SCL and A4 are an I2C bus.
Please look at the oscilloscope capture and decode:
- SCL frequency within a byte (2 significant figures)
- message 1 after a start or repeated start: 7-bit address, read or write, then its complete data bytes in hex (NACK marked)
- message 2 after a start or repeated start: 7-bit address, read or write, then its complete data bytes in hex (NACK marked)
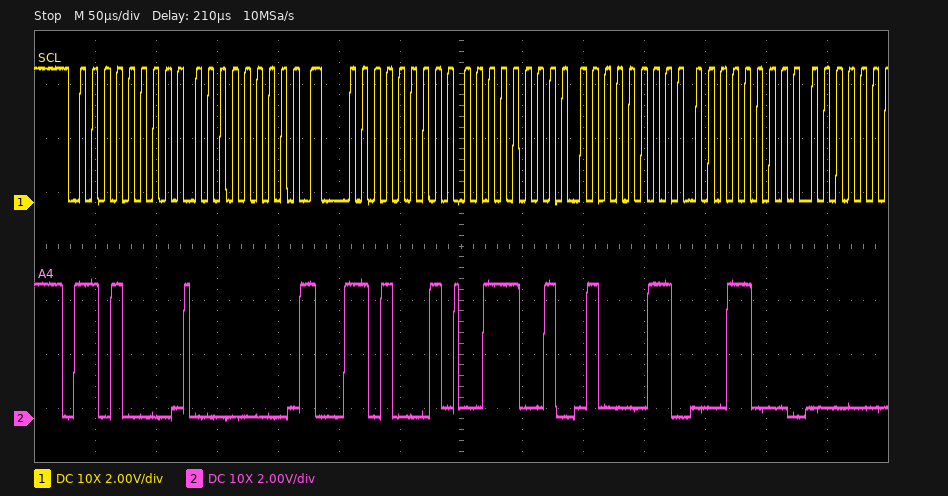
100 kHz
0x68 write: 00
0x68 read: 39 43 18
